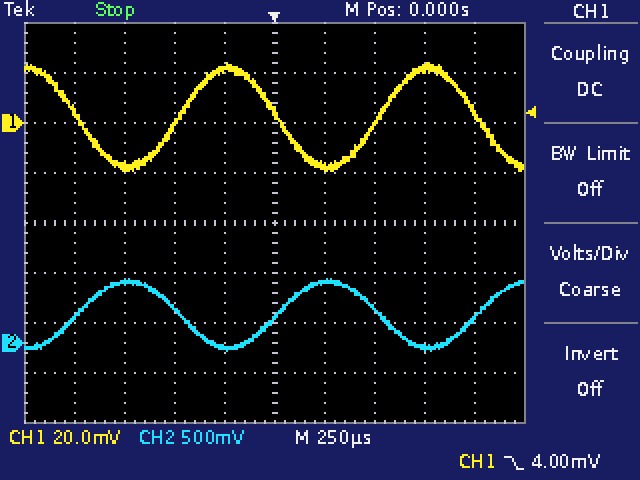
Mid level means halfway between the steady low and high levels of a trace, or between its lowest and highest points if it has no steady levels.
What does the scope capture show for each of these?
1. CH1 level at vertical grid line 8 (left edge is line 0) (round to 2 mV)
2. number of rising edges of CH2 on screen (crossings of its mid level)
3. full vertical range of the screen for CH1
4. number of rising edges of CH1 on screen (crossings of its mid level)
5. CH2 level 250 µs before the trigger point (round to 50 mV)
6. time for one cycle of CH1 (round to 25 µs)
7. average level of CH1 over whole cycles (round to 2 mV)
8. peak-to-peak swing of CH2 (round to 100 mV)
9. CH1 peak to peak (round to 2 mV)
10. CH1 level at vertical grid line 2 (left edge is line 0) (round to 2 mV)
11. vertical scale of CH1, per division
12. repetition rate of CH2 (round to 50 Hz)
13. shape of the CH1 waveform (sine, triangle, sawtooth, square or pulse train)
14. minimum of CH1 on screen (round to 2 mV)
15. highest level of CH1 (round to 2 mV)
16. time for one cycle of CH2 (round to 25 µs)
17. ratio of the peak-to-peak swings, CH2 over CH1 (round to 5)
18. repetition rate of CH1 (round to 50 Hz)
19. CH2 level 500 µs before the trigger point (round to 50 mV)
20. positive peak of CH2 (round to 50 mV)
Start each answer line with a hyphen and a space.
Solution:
- 22 mV
- 3
- 160 mV
- 2
- -50 mV
- 1.000 ms
- 2 mV
- 700 mV
- 44 mV
- -18 mV
- 20 mV
- 1.00 kHz
- sine
- -20 mV
- 24 mV
- 1.000 ms
- 15
- 1.00 kHz
- 350 mV
- 650 mV
